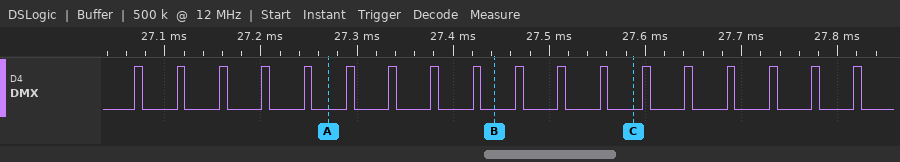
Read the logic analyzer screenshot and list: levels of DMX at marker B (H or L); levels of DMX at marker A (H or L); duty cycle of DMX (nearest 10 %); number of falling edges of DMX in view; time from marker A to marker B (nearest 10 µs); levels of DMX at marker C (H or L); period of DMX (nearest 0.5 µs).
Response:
DMX=L
DMX=L
20 %
18
170 µs
DMX=L
44 µs
